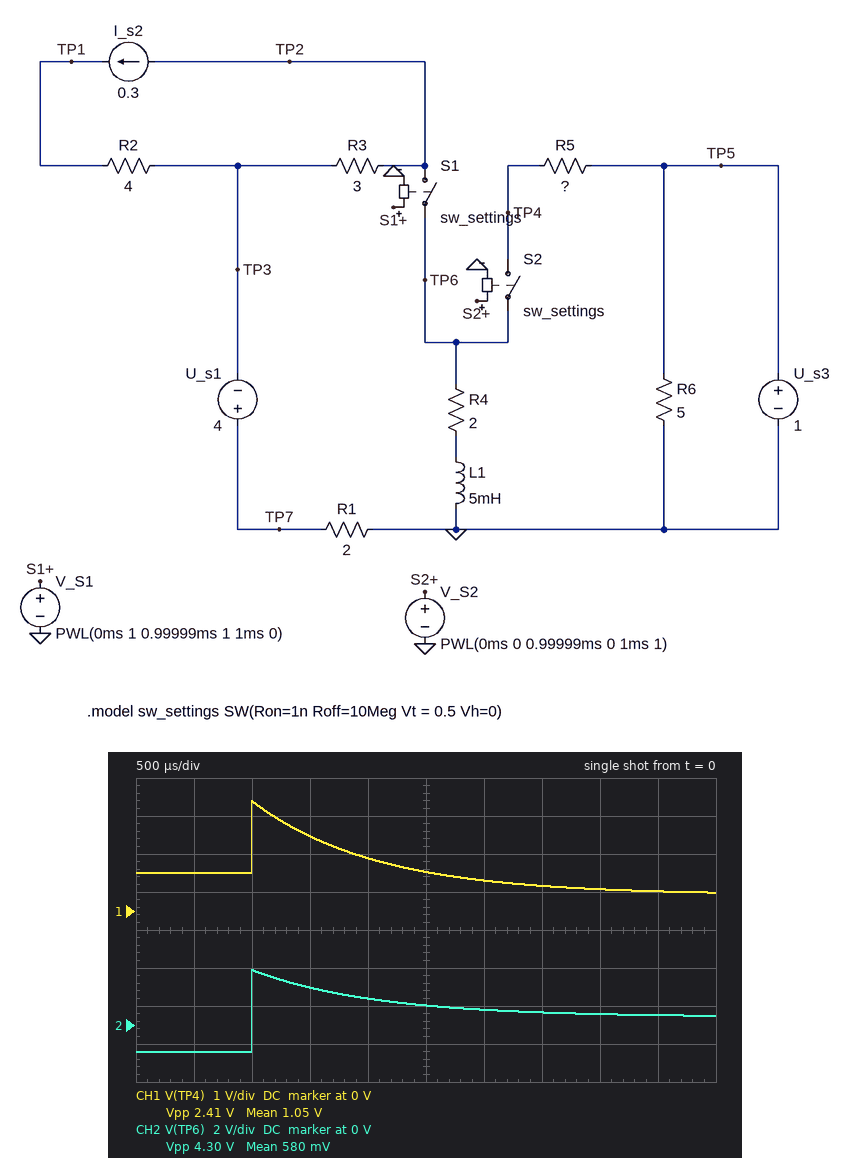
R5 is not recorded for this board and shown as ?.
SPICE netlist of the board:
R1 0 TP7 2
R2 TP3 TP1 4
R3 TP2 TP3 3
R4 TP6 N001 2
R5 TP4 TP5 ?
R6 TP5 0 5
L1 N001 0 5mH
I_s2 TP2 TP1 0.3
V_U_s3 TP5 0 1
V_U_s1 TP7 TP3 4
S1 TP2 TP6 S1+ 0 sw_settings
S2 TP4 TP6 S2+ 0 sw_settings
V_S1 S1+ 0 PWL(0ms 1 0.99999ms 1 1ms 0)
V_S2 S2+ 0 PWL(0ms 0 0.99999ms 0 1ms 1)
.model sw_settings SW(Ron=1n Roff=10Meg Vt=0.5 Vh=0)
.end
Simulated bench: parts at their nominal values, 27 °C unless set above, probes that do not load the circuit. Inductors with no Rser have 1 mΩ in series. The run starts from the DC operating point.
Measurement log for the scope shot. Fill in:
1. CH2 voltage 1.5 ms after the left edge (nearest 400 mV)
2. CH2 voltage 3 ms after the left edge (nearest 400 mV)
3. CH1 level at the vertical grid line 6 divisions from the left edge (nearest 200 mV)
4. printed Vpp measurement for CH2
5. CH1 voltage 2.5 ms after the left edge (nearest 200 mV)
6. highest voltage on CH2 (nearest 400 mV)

2.0 V
800 mV
800 mV
4.30 V
1.0 V
2.8 V
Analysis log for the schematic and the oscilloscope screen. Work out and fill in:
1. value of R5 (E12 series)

2.7 Ω
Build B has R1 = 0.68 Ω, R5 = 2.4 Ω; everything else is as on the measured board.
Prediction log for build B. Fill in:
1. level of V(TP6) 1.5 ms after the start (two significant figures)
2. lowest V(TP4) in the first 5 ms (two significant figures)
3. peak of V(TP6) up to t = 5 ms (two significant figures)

2.1 V
530 mV
3.1 V
